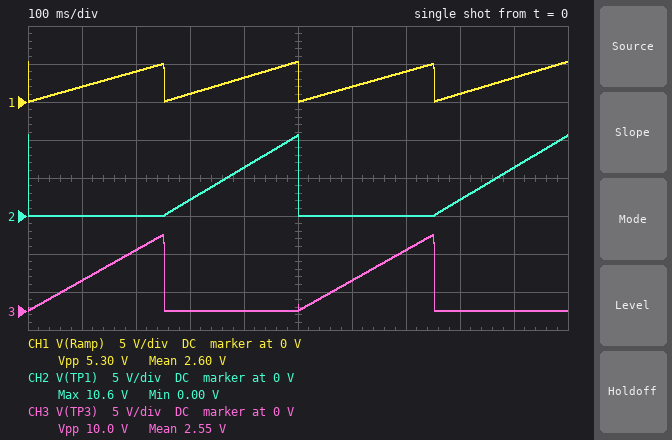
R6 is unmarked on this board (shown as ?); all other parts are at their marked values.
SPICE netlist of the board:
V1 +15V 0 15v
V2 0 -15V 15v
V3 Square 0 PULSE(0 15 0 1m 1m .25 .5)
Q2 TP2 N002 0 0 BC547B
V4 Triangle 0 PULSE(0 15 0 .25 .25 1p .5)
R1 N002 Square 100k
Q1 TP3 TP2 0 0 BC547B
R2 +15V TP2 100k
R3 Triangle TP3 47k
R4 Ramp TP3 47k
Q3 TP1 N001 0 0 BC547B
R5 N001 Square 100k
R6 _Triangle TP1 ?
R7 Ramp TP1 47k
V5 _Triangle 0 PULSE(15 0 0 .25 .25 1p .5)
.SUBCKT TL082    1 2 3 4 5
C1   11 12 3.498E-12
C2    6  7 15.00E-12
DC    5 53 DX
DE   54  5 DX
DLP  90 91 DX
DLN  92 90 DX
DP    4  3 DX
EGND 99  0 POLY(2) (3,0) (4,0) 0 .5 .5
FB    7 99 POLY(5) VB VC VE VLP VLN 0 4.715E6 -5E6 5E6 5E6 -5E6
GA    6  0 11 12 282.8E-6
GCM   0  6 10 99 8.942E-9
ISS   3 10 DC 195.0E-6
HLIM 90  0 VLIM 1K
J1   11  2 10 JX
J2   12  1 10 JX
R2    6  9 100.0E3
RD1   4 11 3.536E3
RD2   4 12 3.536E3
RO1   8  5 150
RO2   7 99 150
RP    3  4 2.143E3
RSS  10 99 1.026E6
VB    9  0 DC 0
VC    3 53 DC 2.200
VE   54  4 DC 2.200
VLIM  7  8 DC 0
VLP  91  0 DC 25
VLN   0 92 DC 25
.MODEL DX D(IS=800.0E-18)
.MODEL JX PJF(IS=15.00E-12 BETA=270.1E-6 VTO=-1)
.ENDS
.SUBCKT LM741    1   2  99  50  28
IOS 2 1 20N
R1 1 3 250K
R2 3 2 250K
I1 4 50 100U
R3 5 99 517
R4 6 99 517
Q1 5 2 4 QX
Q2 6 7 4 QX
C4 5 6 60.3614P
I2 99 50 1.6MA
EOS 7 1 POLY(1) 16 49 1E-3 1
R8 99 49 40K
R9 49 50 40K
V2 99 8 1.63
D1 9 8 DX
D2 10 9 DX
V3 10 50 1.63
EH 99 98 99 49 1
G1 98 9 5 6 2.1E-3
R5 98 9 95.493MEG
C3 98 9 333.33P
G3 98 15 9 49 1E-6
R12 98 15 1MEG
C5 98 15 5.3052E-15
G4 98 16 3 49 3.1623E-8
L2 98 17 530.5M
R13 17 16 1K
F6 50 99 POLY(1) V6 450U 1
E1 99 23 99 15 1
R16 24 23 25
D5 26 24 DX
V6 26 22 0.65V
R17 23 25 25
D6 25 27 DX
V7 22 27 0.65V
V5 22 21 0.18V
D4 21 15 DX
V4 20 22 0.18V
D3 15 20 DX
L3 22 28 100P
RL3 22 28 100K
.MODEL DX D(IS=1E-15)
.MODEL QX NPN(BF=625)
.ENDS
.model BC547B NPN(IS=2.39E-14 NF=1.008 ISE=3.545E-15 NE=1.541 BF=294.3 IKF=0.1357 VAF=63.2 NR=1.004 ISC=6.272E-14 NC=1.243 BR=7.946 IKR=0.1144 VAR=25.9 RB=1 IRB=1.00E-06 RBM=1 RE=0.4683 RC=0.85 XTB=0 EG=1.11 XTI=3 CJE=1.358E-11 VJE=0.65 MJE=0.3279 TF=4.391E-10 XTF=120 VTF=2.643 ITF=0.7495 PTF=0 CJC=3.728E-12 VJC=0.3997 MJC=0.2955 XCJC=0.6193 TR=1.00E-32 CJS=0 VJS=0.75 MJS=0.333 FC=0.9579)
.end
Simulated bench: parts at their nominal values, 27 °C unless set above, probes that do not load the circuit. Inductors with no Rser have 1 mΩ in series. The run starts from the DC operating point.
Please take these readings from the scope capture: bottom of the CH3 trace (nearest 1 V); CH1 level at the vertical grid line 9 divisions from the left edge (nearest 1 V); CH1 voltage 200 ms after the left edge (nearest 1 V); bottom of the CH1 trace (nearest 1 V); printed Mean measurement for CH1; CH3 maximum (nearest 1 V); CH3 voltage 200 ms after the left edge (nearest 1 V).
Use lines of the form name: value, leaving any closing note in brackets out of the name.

bottom of the CH3 trace: 0 V
CH1 level at the vertical grid line 9 divisions from the left edge: 3 V
CH1 voltage 200 ms after the left edge: 4 V
bottom of the CH1 trace: 0 V
printed Mean measurement for CH1: 2.60 V
CH3 maximum: 10 V
CH3 voltage 200 ms after the left edge: 8 V
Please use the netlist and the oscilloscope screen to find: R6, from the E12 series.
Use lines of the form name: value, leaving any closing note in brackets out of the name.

R6, from the E12 series: 39 kΩ
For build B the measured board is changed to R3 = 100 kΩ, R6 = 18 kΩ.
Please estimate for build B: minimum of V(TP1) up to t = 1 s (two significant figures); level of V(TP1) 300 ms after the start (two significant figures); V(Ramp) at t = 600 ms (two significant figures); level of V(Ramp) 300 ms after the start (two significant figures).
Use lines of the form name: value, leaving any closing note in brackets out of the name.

minimum of V(TP1) up to t = 1 s: 8.4 mV
level of V(TP1) 300 ms after the start: 2.5 V
V(Ramp) at t = 600 ms: 1.5 V
level of V(Ramp) 300 ms after the start: 1.3 V
